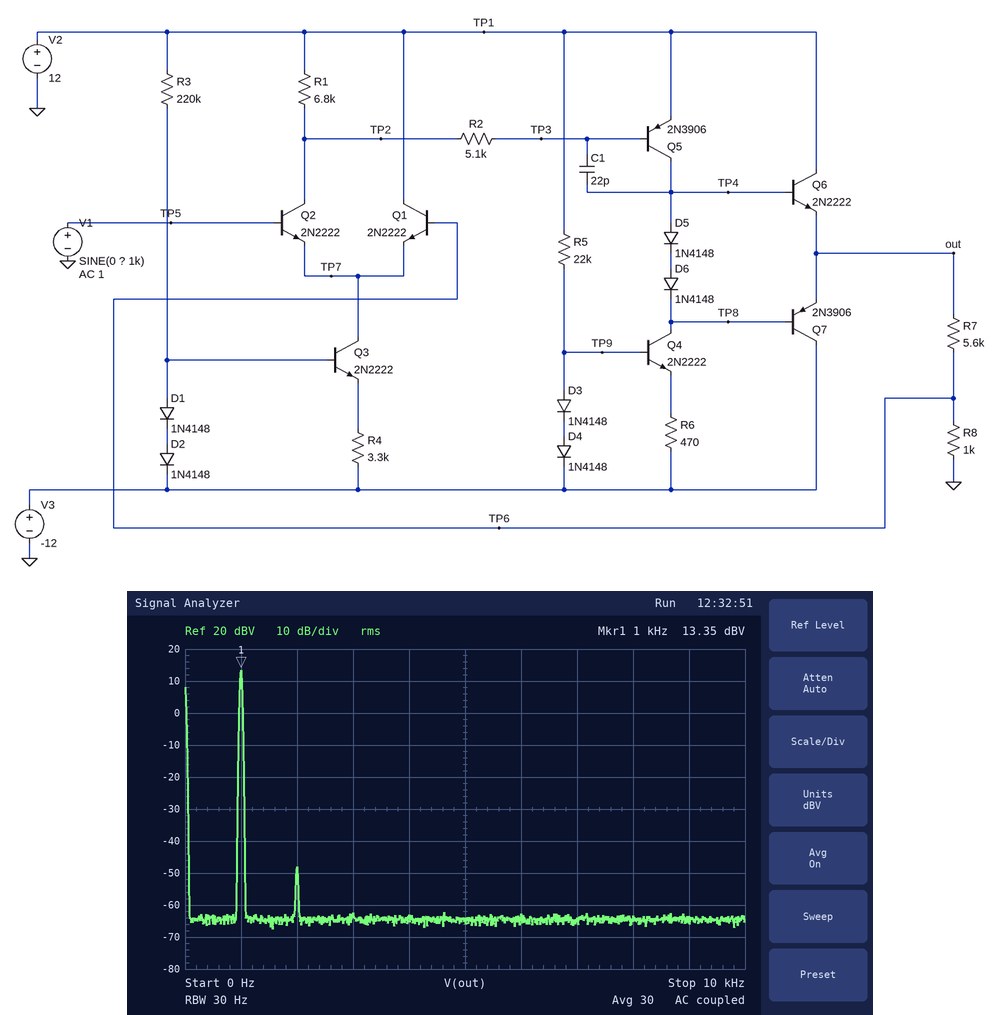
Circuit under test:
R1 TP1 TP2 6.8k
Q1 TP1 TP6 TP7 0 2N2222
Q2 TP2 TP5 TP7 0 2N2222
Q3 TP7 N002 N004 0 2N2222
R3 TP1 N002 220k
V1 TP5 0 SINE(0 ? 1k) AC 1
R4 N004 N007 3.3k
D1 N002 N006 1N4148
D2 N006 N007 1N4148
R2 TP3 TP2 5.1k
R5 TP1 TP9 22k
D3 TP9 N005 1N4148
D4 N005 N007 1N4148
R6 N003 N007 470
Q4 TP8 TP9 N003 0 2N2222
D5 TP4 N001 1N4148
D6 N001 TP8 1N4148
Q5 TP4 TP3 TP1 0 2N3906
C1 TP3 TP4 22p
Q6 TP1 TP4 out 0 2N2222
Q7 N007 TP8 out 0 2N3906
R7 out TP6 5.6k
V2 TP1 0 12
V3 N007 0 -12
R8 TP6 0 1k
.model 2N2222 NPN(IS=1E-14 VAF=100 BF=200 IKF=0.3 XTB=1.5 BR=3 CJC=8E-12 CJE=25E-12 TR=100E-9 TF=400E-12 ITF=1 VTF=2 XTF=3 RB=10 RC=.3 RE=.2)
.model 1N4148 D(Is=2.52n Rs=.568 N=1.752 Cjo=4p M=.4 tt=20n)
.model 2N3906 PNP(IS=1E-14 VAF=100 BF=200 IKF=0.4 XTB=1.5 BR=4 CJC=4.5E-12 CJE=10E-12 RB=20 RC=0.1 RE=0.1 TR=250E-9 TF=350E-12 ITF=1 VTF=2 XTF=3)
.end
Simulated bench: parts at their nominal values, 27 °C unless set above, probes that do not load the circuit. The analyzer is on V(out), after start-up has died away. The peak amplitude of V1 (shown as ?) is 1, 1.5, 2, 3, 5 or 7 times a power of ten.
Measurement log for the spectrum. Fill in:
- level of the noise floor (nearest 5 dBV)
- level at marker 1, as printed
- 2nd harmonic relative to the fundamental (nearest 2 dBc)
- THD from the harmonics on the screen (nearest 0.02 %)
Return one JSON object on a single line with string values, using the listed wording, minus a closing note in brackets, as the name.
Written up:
{"level of the noise floor": "-65 dBV", "level at marker 1, as printed": "13.35 dBV", "2nd harmonic relative to the fundamental": "-62 dBc", "THD from the harmonics on the screen": "0.08 %"}
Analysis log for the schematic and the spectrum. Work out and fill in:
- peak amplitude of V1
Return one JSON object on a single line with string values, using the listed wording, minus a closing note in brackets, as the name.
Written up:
{"peak amplitude of V1": "1 V"}
